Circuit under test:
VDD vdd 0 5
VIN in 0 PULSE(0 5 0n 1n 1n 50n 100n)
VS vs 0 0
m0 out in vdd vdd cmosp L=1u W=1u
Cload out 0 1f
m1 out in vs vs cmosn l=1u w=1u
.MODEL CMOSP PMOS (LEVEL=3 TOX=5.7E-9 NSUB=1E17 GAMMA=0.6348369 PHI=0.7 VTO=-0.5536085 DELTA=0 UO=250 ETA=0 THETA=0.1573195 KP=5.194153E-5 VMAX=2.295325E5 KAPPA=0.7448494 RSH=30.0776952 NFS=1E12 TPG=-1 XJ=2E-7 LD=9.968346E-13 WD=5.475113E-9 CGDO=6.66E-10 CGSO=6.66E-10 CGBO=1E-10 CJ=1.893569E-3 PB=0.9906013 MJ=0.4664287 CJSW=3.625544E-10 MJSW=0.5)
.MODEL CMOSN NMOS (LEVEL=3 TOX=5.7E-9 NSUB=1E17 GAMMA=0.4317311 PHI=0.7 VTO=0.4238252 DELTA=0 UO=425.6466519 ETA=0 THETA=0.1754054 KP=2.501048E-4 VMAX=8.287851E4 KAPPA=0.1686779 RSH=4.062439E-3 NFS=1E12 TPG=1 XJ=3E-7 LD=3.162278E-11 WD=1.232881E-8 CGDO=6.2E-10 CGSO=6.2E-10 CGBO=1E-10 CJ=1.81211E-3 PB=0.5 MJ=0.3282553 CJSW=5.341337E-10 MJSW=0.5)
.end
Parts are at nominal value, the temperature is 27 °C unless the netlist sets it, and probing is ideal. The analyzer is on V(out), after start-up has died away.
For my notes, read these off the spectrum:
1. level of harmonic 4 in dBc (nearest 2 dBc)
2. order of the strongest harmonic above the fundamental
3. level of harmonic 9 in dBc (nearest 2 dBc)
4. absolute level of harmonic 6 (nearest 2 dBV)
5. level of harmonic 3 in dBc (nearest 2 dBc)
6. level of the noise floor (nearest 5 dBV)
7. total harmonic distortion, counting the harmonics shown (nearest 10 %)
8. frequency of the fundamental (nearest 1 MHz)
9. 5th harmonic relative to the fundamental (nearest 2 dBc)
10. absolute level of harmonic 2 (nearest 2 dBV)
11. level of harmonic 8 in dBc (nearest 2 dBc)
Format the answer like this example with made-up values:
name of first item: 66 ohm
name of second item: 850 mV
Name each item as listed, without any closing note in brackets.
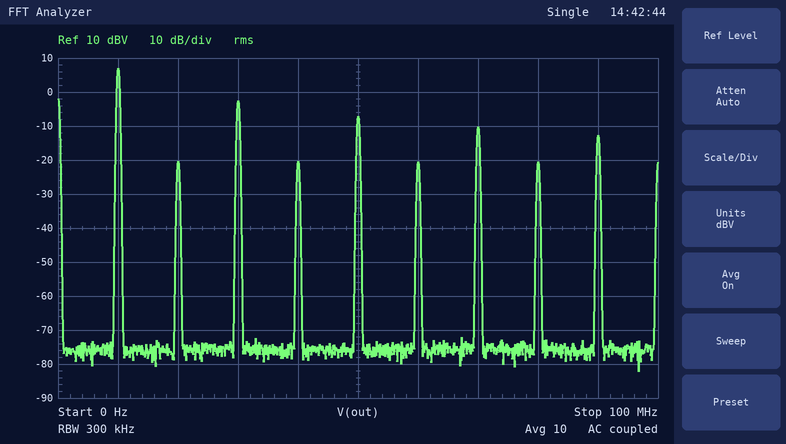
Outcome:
level of harmonic 4 in dBc: -28 dBc
order of the strongest harmonic above the fundamental: 3
level of harmonic 9 in dBc: -20 dBc
absolute level of harmonic 6: -20 dBV
level of harmonic 3 in dBc: -10 dBc
level of the noise floor: -75 dBV
total harmonic distortion, counting the harmonics shown: 40 %
frequency of the fundamental: 10 MHz
5th harmonic relative to the fundamental: -14 dBc
absolute level of harmonic 2: -20 dBV
level of harmonic 8 in dBc: -28 dBc
